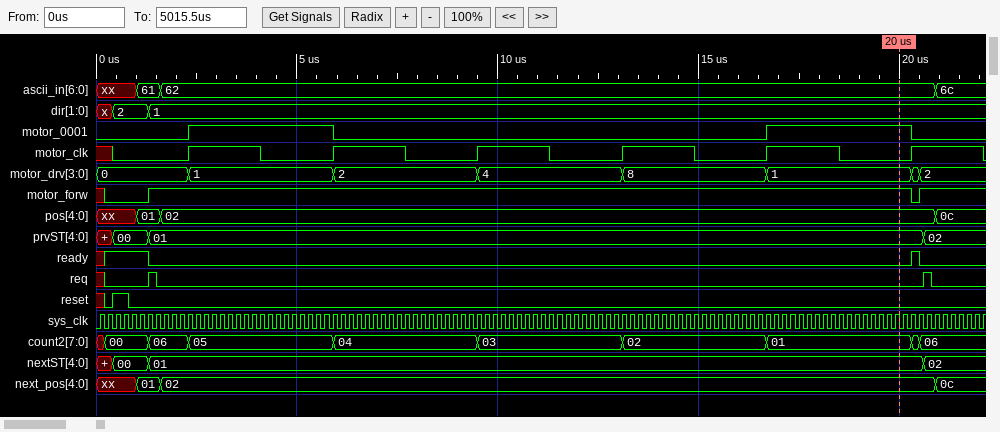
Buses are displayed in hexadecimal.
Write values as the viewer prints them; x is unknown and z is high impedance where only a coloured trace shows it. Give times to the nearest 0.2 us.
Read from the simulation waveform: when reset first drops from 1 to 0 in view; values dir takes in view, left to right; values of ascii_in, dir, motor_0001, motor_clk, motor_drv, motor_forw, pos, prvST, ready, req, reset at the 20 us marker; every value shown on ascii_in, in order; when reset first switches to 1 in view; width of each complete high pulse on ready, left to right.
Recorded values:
0.8 us
x, 2, 1
ascii_in=62, dir=1, motor_0001=1, motor_clk=0, motor_drv=1, motor_forw=1, pos=02, prvST=01, ready=0, req=0, reset=0
xx, 61, 62, 6c
0.4 us
0.2 us
